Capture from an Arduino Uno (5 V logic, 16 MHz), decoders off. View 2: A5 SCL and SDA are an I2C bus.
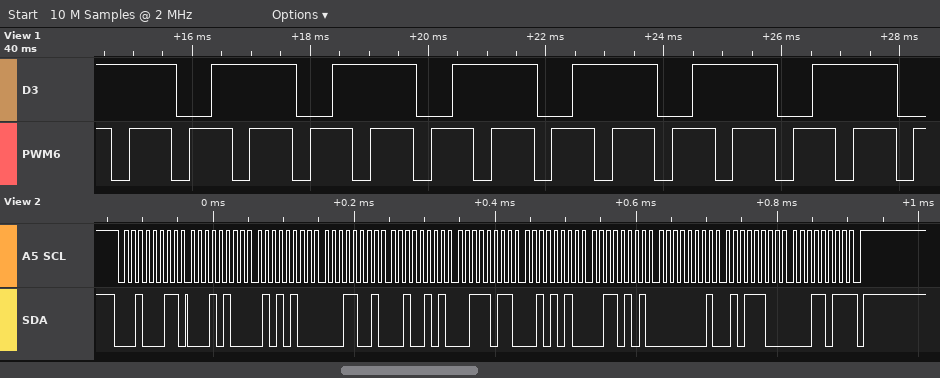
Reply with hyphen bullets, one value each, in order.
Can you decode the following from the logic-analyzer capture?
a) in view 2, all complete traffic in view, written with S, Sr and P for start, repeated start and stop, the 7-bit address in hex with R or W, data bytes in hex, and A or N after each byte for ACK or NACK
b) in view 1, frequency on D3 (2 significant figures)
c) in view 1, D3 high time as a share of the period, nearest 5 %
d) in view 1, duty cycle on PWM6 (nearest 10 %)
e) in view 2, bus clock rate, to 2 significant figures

- S 11R A 14 A 54 A 19 A 25 A 3B A 2A A 35 A 01 A 5C A 1B N P
- 490 Hz
- 70 %
- 70 %
- 100 kHz
